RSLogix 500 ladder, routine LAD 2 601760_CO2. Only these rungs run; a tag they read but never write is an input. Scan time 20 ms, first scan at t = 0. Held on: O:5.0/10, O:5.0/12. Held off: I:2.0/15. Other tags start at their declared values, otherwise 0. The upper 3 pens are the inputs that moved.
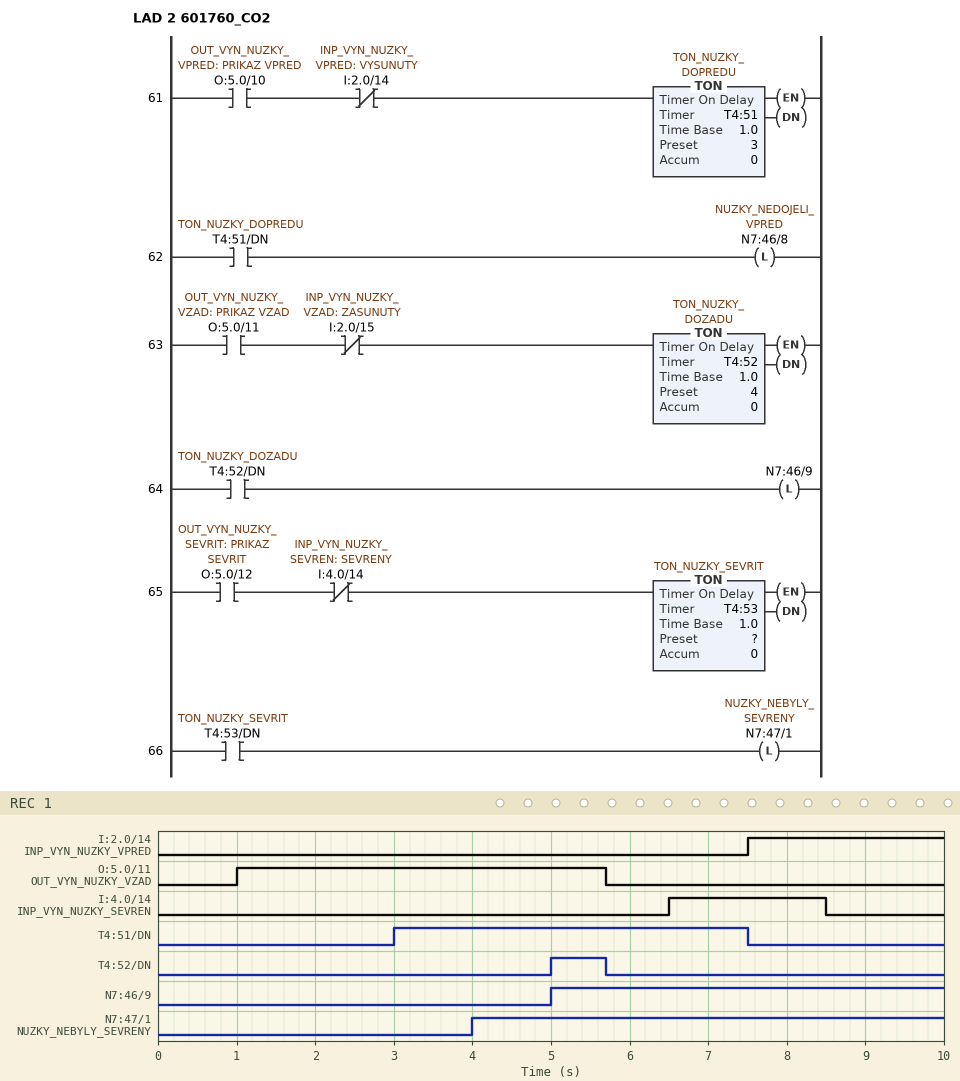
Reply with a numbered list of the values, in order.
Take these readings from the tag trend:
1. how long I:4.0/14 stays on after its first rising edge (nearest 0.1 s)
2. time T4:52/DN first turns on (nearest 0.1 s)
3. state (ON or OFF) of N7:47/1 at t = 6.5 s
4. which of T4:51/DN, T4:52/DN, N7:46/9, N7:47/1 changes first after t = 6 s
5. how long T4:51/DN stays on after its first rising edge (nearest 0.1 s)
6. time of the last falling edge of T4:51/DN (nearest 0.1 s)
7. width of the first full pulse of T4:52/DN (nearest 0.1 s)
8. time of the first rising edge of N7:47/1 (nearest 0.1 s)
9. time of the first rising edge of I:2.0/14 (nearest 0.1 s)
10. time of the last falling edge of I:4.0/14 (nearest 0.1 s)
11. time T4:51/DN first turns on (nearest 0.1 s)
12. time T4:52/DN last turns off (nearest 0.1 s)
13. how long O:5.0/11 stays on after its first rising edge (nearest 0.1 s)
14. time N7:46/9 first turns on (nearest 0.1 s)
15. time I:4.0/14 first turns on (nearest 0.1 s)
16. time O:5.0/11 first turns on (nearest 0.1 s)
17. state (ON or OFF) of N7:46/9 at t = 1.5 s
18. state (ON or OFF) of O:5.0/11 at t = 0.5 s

1. 2.0 s
2. 5.0 s
3. ON
4. T4:51/DN
5. 4.5 s
6. 7.5 s
7. 0.7 s
8. 4.0 s
9. 7.5 s
10. 8.5 s
11. 3.0 s
12. 5.7 s
13. 4.7 s
14. 5.0 s
15. 6.5 s
16. 1.0 s
17. OFF
18. OFF
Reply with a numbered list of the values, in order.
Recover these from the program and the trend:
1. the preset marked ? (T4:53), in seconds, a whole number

1. 4 s
